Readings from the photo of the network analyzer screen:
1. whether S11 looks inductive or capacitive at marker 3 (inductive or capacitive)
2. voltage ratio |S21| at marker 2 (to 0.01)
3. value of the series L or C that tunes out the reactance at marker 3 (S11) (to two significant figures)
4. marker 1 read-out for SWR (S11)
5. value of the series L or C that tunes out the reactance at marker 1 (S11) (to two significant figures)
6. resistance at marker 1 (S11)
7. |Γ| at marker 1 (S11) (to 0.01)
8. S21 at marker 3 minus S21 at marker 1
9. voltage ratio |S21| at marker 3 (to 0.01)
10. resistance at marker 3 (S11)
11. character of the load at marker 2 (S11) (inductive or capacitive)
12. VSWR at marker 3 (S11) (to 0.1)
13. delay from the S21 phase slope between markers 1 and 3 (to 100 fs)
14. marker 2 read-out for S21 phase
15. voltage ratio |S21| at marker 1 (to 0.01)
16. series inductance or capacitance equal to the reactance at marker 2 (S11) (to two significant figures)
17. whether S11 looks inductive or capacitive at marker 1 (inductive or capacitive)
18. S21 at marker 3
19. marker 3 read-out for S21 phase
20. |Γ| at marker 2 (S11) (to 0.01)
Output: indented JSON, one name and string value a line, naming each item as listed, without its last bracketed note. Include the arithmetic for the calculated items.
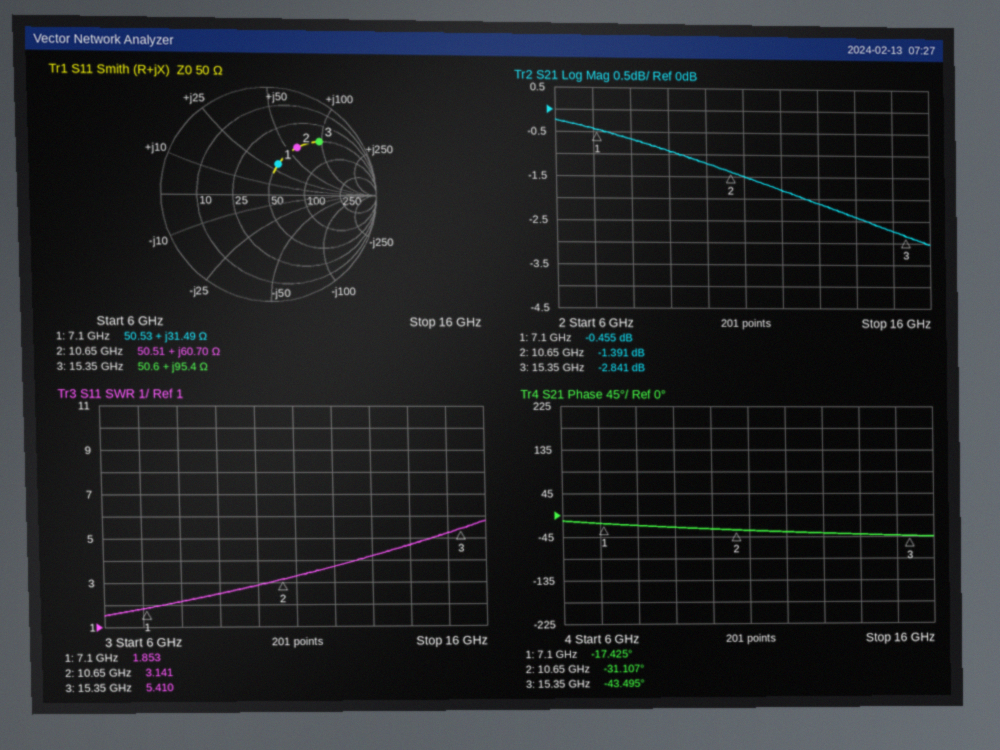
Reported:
{
  "whether S11 looks inductive or capacitive at marker 3": "inductive",
  "voltage ratio |S21| at marker 2": "10^(-1.391/20) ≈ 0.85",
  "value of the series L or C that tunes out the reactance at marker 3 (S11)": "C = 1/(2π × 15.35 GHz × 95.4 Ω) ≈ 109 fF, so 110 fF to two significant figures",
  "marker 1 read-out for SWR": "1.853",
  "value of the series L or C that tunes out the reactance at marker 1 (S11)": "C = 1/(2π × 7.1 GHz × 31.49 Ω) ≈ 712 fF, so 710 fF to two significant figures",
  "resistance at marker 1": "50.53 Ω",
  "|Γ| at marker 1 (S11)": "0.30",
  "S21 at marker 3 minus S21 at marker 1": "-2.841 − (-0.455) = -2.386 dB",
  "voltage ratio |S21| at marker 3": "10^(-2.841/20) ≈ 0.72",
  "resistance at marker 3": "50.6 Ω",
  "character of the load at marker 2 (S11)": "inductive",
  "VSWR at marker 3 (S11)": "5.4",
  "delay from the S21 phase slope between markers 1 and 3": "−(-43.495° − (-17.425°))/(360° × 8.25 GHz) ≈ 8.8 ps",
  "marker 2 read-out for S21 phase": "-31.107°",
  "voltage ratio |S21| at marker 1": "10^(-0.455/20) ≈ 0.95",
  "series inductance or capacitance equal to the reactance at marker 2 (S11)": "L = 60.7 Ω/(2π × 10.65 GHz) ≈ 907 pH, so 910 pH to two significant figures",
  "whether S11 looks inductive or capacitive at marker 1": "inductive",
  "S21 at marker 3": "-2.841 dB",
  "marker 3 read-out for S21 phase": "-43.495°",
  "|Γ| at marker 2 (S11)": "0.52"
}
